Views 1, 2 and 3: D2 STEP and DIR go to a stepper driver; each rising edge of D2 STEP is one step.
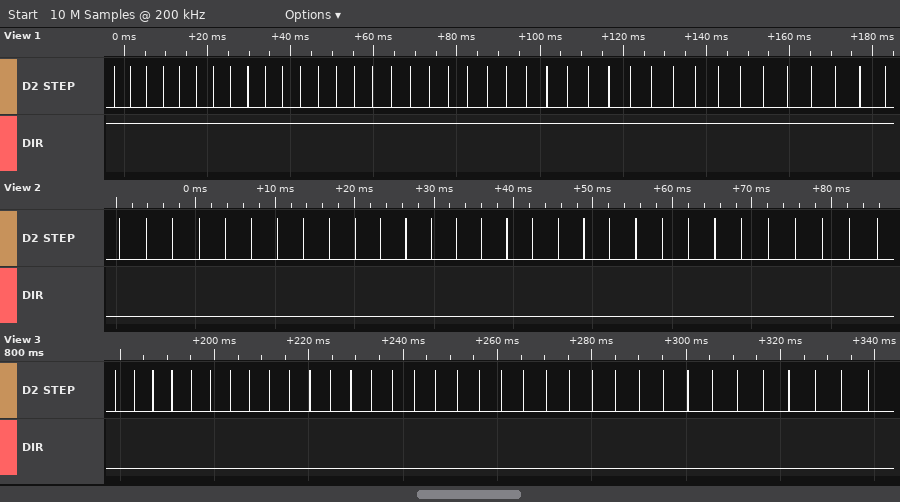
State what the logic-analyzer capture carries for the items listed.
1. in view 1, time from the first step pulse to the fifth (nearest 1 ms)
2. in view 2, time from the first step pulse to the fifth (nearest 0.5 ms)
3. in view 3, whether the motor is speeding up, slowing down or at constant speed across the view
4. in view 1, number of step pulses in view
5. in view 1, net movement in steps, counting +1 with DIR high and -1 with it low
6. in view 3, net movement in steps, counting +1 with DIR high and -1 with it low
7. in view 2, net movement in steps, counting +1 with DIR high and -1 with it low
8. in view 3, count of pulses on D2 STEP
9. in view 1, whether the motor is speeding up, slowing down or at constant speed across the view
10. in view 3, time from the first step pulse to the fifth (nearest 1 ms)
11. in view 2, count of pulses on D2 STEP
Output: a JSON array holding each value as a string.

["16 ms", "13.5 ms", "slowing down", "40", "+40", "-35", "-30", "35", "slowing down", "16 ms", "30"]
